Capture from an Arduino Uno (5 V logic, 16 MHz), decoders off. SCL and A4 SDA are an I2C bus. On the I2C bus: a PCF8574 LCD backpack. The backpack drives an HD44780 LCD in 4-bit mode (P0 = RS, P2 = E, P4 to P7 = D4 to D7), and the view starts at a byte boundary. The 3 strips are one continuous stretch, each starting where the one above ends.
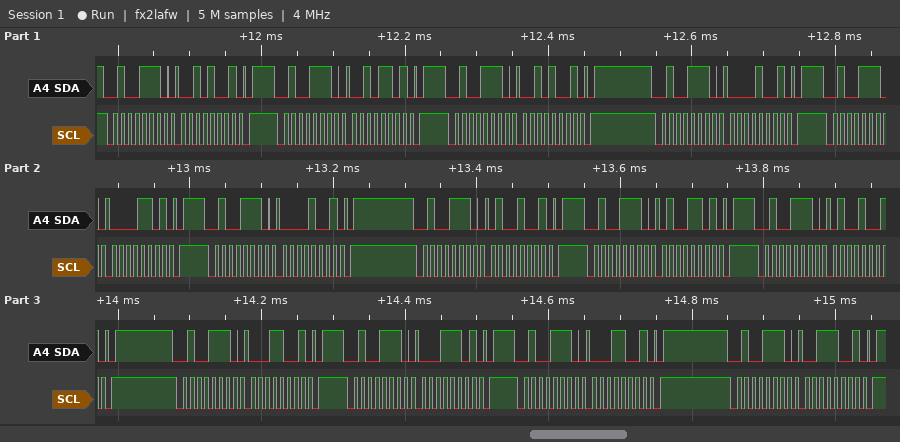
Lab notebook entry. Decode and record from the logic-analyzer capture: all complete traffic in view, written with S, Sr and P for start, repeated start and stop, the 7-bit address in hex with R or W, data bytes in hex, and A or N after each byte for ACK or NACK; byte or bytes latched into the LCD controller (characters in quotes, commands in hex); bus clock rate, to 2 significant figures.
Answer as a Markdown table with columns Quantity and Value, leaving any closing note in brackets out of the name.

| Quantity | Value |
|---|---|
| all complete traffic in view, written with S, Sr and P for start, repeated start and stop, the 7-bit address in hex with R or W, data bytes in hex, and A or N after each byte for ACK or NACK | S 27W A 29 A P S 27W A 2D A P S 27W A 29 A P S 27W A 09 A P S 27W A 0D A P S 27W A 09 A P S 27W A 49 A P S 27W A 4D A P S 27W A 49 A P S 27W A 19 A P S 27W A 1D A P S 27W A 19 A P S 27W A 39 A P |
| byte or bytes latched into the LCD controller | ' ' 'A' |
| bus clock rate, to 2 significant figures | 100 kHz |
